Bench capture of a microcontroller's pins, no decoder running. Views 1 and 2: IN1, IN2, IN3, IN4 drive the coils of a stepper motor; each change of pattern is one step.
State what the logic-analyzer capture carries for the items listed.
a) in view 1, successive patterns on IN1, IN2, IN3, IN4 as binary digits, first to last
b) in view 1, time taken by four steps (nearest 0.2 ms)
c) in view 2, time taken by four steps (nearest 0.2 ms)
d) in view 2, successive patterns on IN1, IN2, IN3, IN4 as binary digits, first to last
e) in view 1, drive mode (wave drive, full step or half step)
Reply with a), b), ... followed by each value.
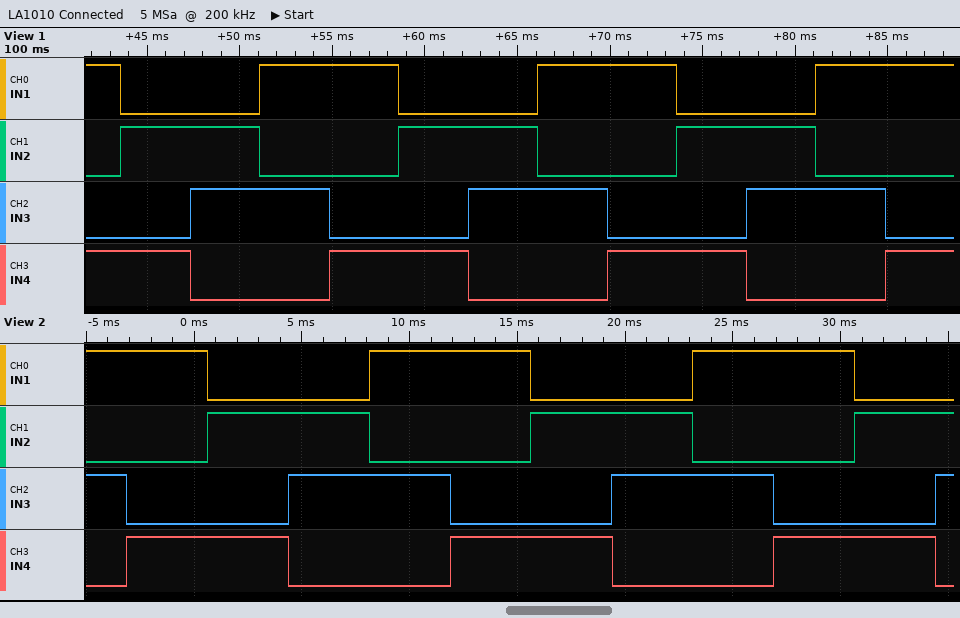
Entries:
a) 1001 0101 0110 1010 1001 0101 0110 1010 1001 0101 0110 1010 1001
b) 15.0 ms
c) 15.0 ms
d) 1010 1001 0101 0110 1010 1001 0101 0110 1010 1001 0101 0110
e) full step
